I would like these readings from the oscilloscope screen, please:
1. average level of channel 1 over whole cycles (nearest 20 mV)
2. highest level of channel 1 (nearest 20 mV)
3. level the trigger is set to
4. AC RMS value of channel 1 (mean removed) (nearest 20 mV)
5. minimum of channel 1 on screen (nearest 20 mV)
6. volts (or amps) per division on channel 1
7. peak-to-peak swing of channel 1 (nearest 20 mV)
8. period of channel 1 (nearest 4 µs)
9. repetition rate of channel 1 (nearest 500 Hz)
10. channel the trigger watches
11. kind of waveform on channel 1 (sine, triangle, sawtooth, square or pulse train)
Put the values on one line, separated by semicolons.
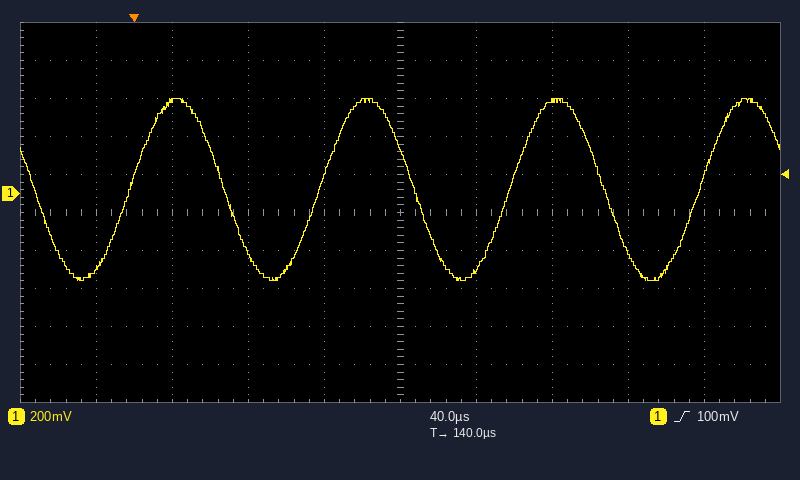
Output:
20 mV; 500 mV; 100 mV; 340 mV; -460 mV; 200 mV; 960 mV; 100 µs; 10.0 kHz; channel 1; sine
